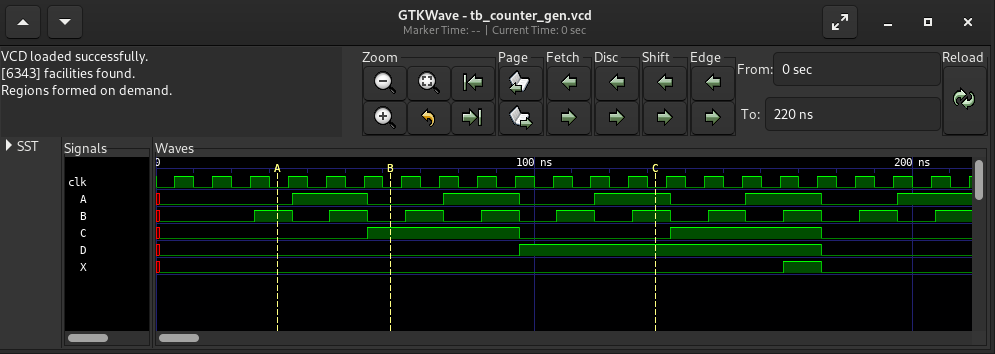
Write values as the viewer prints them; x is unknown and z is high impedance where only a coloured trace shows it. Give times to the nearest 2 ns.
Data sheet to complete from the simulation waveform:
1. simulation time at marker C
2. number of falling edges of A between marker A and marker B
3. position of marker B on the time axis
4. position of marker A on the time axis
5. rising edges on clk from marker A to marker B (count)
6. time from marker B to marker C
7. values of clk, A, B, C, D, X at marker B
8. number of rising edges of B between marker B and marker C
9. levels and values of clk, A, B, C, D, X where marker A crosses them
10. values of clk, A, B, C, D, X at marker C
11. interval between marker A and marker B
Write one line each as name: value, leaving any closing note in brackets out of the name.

simulation time at marker C: 132 ns
number of falling edges of A between marker A and marker B: 1
position of marker B on the time axis: 62 ns
position of marker A on the time axis: 32 ns
rising edges on clk from marker A to marker B: 3
time from marker B to marker C: 70 ns
values of clk, A, B, C, D, X at marker B: clk=0, A=0, B=0, C=1, D=0, X=0
number of rising edges of B between marker B and marker C: 4
levels and values of clk, A, B, C, D, X where marker A crosses them: clk=0, A=0, B=1, C=0, D=0, X=0
values of clk, A, B, C, D, X at marker C: clk=0, A=1, B=1, C=0, D=1, X=0
interval between marker A and marker B: 30 ns
